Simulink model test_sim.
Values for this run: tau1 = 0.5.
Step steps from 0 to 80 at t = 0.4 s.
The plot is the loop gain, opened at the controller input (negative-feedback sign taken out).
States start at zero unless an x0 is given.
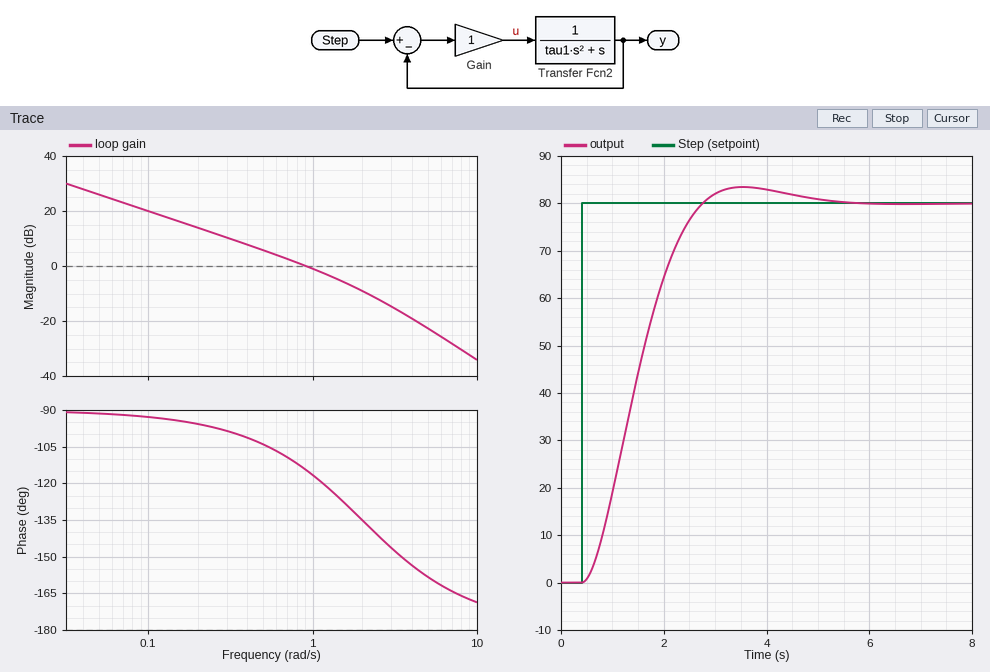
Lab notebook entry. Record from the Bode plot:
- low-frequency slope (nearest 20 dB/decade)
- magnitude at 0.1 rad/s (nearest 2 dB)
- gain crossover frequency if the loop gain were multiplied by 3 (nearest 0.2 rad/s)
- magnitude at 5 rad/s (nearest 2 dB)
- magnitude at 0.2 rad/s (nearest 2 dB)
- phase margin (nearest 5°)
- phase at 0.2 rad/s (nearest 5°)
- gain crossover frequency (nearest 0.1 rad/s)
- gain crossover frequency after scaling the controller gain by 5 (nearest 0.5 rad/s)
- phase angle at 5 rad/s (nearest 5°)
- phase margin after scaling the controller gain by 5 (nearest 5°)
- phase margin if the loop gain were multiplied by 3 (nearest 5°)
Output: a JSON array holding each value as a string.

["-20 dB/decade", "20 dB", "2.0 rad/s", "-22 dB", "14 dB", "65°", "-95°", "0.9 rad/s", "3.0 rad/s", "-160°", "35°", "45°"]
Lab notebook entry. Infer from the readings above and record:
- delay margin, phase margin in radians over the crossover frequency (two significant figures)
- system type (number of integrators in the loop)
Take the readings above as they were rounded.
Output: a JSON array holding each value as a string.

["1.3 s", "1"]
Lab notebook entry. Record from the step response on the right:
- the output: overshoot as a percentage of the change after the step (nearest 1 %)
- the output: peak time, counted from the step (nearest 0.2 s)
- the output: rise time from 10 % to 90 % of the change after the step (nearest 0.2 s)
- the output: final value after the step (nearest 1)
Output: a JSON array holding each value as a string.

["4 %", "3.2 s", "1.6 s", "80"]
